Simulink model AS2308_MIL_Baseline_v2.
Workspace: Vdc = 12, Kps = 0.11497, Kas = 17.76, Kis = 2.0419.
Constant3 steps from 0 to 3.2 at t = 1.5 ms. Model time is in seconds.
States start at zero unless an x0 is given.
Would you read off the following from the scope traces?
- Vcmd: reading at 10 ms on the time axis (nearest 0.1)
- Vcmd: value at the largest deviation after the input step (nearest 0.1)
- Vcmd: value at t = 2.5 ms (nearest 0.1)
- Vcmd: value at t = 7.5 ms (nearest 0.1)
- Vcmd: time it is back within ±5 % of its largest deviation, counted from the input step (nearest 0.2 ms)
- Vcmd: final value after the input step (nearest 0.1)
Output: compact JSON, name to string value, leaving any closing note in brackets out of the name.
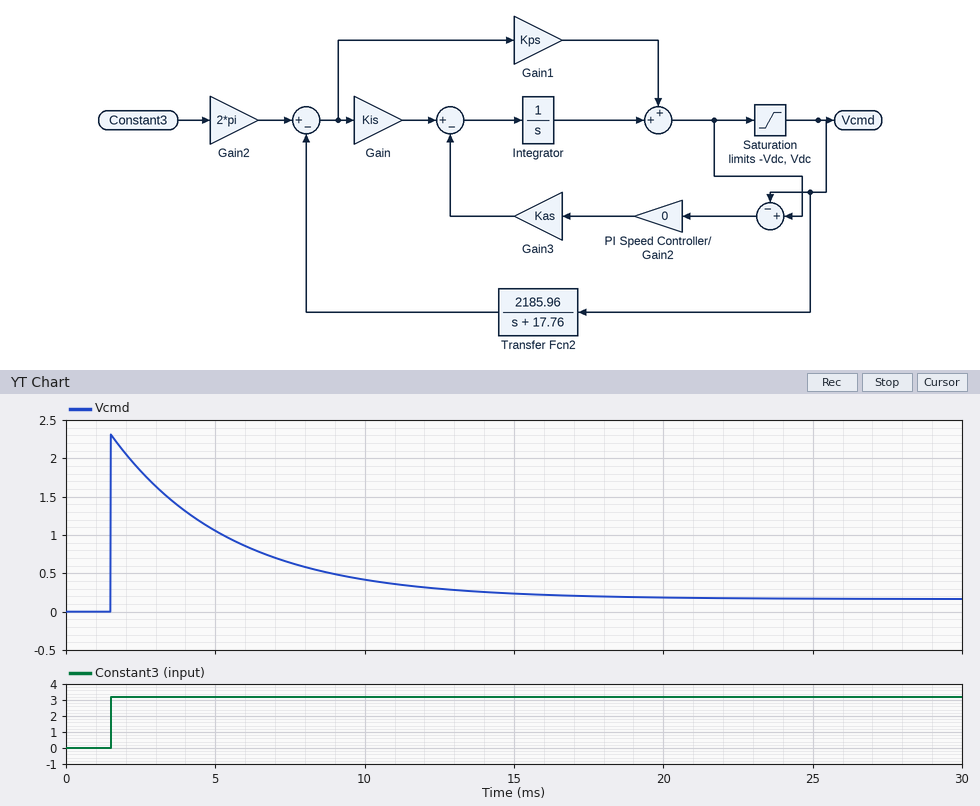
{"Vcmd: reading at 10 ms on the time axis": "0.4", "Vcmd: value at the largest deviation after the input step": "2.3", "Vcmd: value at t = 2.5 ms": "1.8", "Vcmd: value at t = 7.5 ms": "0.6", "Vcmd: time it is back within ±5 % of its largest deviation, counted from the input step": "11.6 ms", "Vcmd: final value after the input step": "0.2"}
